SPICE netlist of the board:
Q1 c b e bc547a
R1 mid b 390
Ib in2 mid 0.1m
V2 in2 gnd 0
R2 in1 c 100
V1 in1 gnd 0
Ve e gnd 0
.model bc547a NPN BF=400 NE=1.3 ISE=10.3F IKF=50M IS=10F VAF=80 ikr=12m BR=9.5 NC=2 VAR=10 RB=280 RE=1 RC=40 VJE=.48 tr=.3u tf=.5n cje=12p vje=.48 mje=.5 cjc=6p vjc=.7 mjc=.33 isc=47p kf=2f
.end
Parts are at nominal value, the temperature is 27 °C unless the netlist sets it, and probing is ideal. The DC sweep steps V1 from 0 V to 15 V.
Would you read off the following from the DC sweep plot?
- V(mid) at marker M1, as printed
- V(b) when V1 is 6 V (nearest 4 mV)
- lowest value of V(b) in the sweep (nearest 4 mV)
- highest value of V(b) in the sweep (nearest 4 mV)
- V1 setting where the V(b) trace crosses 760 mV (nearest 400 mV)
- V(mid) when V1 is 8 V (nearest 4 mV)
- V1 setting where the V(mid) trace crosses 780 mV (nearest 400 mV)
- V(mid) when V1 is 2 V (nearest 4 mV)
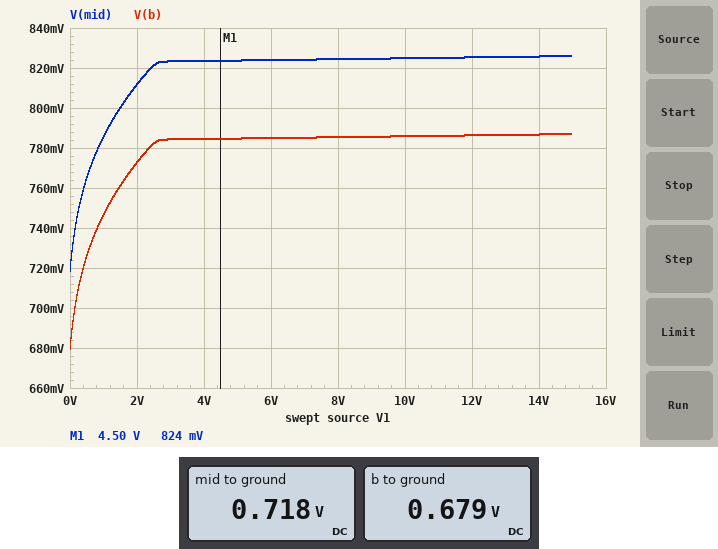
824 mV
784 mV
680 mV
788 mV
1.6 V
824 mV
800 mV
812 mV
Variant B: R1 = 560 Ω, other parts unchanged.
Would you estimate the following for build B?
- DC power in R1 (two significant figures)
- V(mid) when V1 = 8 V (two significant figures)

5.6 µW
840 mV
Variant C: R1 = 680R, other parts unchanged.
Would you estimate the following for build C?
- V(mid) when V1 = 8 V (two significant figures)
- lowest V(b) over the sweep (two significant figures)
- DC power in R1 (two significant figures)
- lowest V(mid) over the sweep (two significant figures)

850 mV
680 mV
6.8 µW
750 mV
